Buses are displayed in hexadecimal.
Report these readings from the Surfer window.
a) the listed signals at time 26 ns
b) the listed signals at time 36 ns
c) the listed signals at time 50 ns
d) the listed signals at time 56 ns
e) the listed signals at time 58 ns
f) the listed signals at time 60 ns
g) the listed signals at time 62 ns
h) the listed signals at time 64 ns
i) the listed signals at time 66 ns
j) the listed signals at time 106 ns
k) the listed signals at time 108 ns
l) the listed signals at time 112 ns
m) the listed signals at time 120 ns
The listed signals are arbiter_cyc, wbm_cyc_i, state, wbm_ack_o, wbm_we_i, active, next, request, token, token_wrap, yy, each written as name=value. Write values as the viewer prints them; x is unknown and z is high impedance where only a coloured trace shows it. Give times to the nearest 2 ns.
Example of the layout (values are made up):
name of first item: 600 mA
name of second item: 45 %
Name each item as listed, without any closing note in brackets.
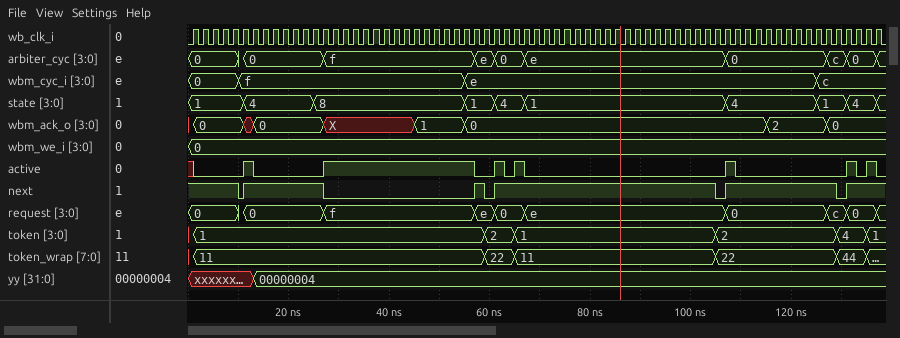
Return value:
the listed signals at time 26 ns: arbiter_cyc=0, wbm_cyc_i=f, state=8, wbm_ack_o=0, wbm_we_i=0, active=0, next=1, request=0, token=1, token_wrap=11, yy=00000004
the listed signals at time 36 ns: arbiter_cyc=f, wbm_cyc_i=f, state=8, wbm_ack_o=X, wbm_we_i=0, active=1, next=0, request=f, token=1, token_wrap=11, yy=00000004
the listed signals at time 50 ns: arbiter_cyc=f, wbm_cyc_i=f, state=8, wbm_ack_o=1, wbm_we_i=0, active=1, next=0, request=f, token=1, token_wrap=11, yy=00000004
the listed signals at time 56 ns: arbiter_cyc=f, wbm_cyc_i=e, state=1, wbm_ack_o=0, wbm_we_i=0, active=1, next=0, request=f, token=1, token_wrap=11, yy=00000004
the listed signals at time 58 ns: arbiter_cyc=e, wbm_cyc_i=e, state=1, wbm_ack_o=0, wbm_we_i=0, active=0, next=1, request=e, token=1, token_wrap=11, yy=00000004
the listed signals at time 60 ns: arbiter_cyc=e, wbm_cyc_i=e, state=1, wbm_ack_o=0, wbm_we_i=0, active=0, next=0, request=e, token=2, token_wrap=22, yy=00000004
the listed signals at time 62 ns: arbiter_cyc=0, wbm_cyc_i=e, state=4, wbm_ack_o=0, wbm_we_i=0, active=1, next=1, request=0, token=2, token_wrap=22, yy=00000004
the listed signals at time 64 ns: arbiter_cyc=0, wbm_cyc_i=e, state=4, wbm_ack_o=0, wbm_we_i=0, active=0, next=1, request=0, token=2, token_wrap=22, yy=00000004
the listed signals at time 66 ns: arbiter_cyc=0, wbm_cyc_i=e, state=4, wbm_ack_o=0, wbm_we_i=0, active=1, next=1, request=0, token=1, token_wrap=11, yy=00000004
the listed signals at time 106 ns: arbiter_cyc=e, wbm_cyc_i=e, state=1, wbm_ack_o=0, wbm_we_i=0, active=0, next=0, request=e, token=2, token_wrap=22, yy=00000004
the listed signals at time 108 ns: arbiter_cyc=0, wbm_cyc_i=e, state=4, wbm_ack_o=0, wbm_we_i=0, active=1, next=1, request=0, token=2, token_wrap=22, yy=00000004
the listed signals at time 112 ns: arbiter_cyc=0, wbm_cyc_i=e, state=4, wbm_ack_o=0, wbm_we_i=0, active=0, next=1, request=0, token=2, token_wrap=22, yy=00000004
the listed signals at time 120 ns: arbiter_cyc=0, wbm_cyc_i=e, state=4, wbm_ack_o=2, wbm_we_i=0, active=0, next=1, request=0, token=2, token_wrap=22, yy=00000004
